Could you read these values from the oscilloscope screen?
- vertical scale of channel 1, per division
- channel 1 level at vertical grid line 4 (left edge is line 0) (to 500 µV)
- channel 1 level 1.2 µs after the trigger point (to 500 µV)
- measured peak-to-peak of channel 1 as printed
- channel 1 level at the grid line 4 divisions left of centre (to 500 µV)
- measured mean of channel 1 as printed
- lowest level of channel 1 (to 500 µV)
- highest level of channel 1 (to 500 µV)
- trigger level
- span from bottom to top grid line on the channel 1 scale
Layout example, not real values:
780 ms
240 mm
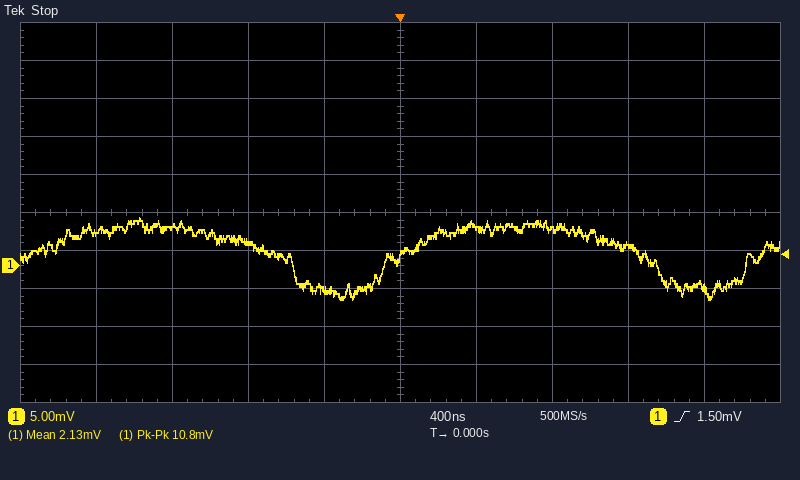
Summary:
5 mV
-3.0 mV
3.0 mV
10.8 mV
4.5 mV
2.13 mV
-4.5 mV
6.5 mV
1.50 mV
50 mV
